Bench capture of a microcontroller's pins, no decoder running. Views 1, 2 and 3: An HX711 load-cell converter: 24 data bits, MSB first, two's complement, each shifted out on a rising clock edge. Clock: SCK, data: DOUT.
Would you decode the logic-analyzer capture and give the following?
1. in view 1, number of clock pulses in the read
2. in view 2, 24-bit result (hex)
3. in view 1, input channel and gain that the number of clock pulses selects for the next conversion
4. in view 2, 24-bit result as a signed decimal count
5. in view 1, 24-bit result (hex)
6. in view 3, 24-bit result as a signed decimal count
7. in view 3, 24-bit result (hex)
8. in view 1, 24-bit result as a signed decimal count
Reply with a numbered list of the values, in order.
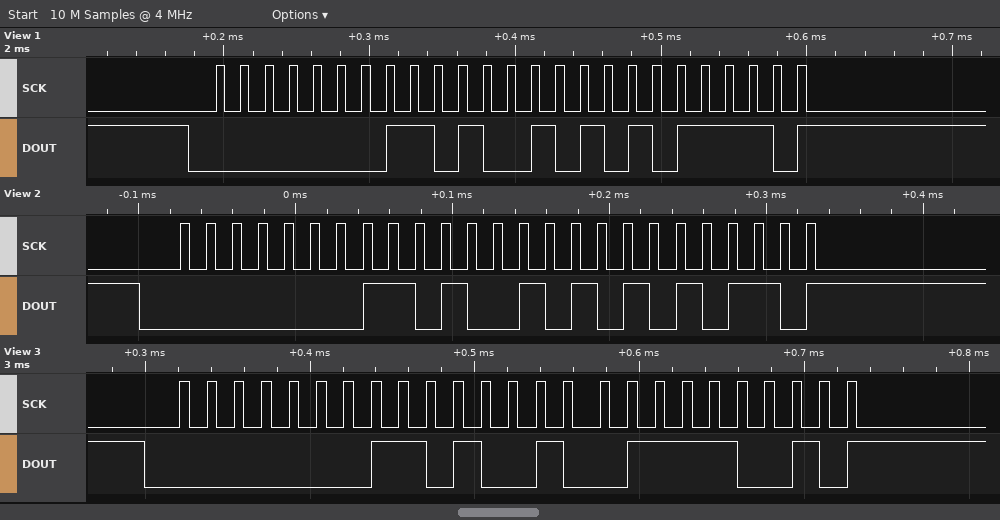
1. 25
2. 0x01A556
3. channel A, gain 128
4. 107862
5. 0x01A55E
6. 107762
7. 0x01A4F2
8. 107870
